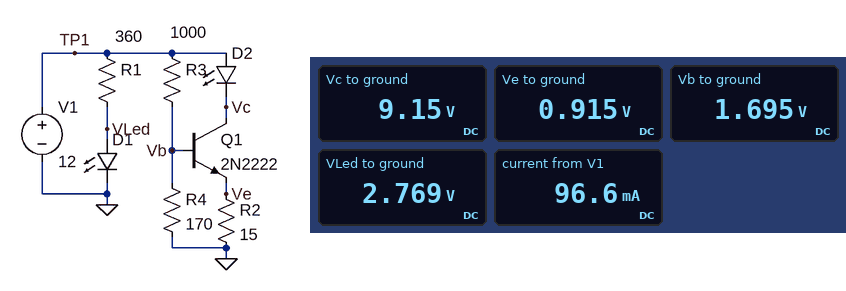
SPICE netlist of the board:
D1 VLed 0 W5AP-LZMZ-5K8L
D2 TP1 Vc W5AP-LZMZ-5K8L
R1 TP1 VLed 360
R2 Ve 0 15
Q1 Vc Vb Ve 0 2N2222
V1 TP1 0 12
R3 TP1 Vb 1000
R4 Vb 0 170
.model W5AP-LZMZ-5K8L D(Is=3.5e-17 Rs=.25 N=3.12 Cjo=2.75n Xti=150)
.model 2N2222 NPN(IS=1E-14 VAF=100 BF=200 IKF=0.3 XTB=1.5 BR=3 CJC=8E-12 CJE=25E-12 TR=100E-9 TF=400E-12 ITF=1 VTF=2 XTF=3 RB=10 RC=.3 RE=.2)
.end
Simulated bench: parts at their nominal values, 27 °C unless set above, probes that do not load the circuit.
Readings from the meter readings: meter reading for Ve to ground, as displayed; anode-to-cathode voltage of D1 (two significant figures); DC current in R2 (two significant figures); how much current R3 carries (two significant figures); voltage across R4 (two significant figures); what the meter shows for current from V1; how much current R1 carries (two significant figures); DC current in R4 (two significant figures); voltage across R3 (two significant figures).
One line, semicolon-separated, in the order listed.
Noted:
0.915 V; 2.8 V; 61 mA; 10 mA; 1.7 V; 96.6 mA; 26 mA; 10 mA; 10 V
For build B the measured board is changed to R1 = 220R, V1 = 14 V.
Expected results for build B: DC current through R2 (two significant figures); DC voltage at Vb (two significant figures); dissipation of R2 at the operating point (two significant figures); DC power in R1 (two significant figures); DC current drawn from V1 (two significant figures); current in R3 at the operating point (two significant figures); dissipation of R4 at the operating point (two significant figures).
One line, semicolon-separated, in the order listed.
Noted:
79 mA; 2.0 V; 93 mW; 570 mW; 140 mA; 12 mA; 23 mW
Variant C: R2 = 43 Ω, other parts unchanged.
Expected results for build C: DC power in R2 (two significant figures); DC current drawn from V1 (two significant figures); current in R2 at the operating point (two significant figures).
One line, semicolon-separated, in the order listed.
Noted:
23 mW; 59 mA; 23 mA
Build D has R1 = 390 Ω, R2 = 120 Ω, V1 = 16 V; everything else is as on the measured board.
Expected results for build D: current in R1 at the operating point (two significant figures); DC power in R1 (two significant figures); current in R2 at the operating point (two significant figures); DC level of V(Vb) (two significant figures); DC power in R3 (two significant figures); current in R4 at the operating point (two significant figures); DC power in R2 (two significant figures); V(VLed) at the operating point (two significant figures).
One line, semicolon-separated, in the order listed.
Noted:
34 mA; 450 mW; 13 mA; 2.3 V; 190 mW; 14 mA; 21 mW; 2.8 V
